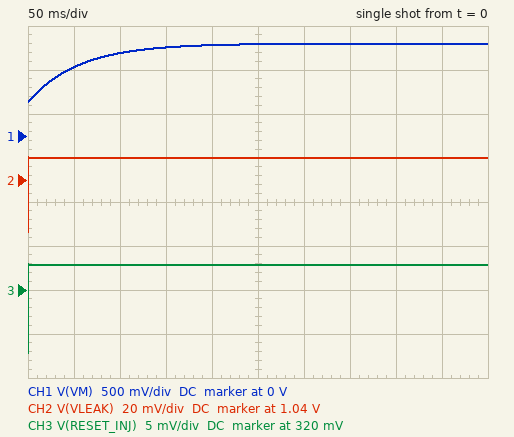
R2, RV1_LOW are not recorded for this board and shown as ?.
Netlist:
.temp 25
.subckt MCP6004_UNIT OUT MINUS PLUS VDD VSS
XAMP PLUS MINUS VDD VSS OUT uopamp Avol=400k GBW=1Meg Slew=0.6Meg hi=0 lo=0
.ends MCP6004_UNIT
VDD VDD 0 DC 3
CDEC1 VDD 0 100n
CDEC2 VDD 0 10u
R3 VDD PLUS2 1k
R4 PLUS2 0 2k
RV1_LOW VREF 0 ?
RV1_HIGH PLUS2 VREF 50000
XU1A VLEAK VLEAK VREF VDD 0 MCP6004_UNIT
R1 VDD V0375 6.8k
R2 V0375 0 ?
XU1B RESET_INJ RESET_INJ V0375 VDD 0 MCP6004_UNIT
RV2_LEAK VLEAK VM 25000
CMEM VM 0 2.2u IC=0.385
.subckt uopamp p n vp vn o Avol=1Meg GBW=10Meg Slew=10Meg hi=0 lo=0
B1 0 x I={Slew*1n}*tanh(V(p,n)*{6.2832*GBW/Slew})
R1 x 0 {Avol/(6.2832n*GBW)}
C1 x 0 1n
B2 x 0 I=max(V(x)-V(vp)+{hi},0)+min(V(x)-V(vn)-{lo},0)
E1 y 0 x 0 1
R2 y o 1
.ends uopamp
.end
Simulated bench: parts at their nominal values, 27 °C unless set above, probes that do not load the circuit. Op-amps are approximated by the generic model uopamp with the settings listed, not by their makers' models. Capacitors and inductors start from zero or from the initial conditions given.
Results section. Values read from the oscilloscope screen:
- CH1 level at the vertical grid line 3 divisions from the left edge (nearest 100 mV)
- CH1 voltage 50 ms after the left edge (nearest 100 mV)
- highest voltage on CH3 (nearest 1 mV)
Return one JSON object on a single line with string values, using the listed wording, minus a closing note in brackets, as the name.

{"CH1 level at the vertical grid line 3 divisions from the left edge": "1.0 V", "CH1 voltage 50 ms after the left edge": "800 mV", "highest voltage on CH3": "323 mV"}
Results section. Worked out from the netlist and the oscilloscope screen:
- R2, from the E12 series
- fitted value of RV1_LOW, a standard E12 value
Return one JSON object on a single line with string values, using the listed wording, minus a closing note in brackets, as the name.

{"R2, from the E12 series": "820 Ω", "fitted value of RV1_LOW, a standard E12 value": "56 kΩ"}
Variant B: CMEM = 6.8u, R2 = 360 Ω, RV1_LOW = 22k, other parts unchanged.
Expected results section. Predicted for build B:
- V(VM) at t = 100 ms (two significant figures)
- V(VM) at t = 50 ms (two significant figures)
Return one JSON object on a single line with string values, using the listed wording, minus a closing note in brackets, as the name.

{"V(VM) at t = 100 ms": "480 mV", "V(VM) at t = 50 ms": "440 mV"}
